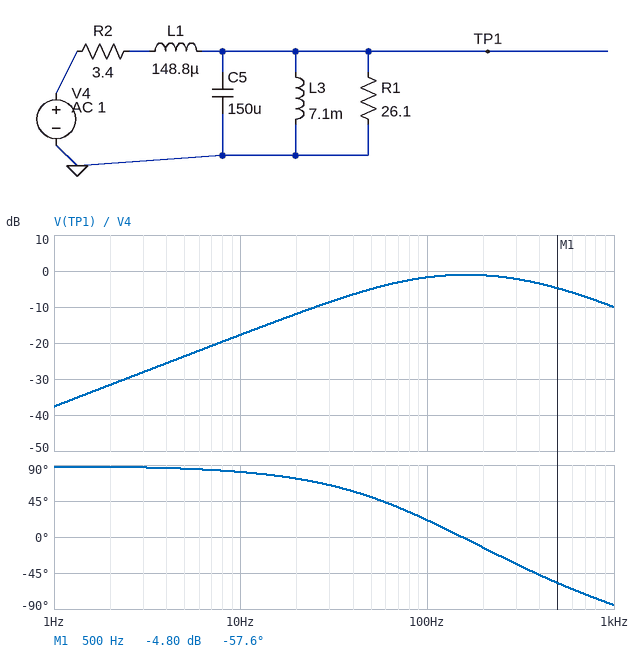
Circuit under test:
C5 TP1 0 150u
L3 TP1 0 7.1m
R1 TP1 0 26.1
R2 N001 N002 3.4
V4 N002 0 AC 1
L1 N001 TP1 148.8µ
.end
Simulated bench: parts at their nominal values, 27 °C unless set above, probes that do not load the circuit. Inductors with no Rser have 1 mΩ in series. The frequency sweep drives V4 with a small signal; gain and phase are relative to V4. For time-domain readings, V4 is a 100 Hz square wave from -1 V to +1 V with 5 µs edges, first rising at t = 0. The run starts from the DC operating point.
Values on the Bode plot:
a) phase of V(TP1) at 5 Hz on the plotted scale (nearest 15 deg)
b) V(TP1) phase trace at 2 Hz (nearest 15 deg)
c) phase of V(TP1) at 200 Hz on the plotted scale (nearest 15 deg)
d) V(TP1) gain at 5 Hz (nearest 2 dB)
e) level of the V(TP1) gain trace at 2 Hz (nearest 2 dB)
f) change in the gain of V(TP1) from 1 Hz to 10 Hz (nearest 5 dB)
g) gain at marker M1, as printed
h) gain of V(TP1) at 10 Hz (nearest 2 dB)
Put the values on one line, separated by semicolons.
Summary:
90 deg; 90 deg; -15 deg; -24 dB; -32 dB; 20 dB; -4.80 dB; -18 dB
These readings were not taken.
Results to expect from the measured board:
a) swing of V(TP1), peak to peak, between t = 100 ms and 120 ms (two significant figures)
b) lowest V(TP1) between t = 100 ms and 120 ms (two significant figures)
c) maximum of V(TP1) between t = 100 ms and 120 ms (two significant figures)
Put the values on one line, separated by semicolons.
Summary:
2.5 V; -1.3 V; 1.3 V
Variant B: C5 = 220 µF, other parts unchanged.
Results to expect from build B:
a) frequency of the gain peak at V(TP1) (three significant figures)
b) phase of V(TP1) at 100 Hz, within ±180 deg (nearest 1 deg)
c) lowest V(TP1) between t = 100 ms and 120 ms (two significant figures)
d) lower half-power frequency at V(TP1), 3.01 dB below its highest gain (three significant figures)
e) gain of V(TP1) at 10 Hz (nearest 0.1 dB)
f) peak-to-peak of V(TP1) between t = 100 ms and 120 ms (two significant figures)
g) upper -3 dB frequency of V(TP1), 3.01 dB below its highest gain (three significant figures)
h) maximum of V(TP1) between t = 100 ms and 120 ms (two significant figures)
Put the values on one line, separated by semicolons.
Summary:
131 Hz; 14 deg; -1.2 V; 55.5 Hz; -17.7 dB; 2.4 V; 310 Hz; 1.2 V
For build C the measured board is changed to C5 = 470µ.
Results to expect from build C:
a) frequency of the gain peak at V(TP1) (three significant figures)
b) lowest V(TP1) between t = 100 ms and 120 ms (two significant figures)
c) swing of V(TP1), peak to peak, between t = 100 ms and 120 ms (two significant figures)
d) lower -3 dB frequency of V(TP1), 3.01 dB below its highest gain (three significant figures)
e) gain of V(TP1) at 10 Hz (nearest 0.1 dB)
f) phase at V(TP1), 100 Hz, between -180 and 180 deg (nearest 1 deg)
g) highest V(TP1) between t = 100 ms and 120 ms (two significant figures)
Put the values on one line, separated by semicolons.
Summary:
88.4 Hz; -1.0 V; 2.1 V; 47.8 Hz; -17.6 dB; -12 deg; 1.0 V
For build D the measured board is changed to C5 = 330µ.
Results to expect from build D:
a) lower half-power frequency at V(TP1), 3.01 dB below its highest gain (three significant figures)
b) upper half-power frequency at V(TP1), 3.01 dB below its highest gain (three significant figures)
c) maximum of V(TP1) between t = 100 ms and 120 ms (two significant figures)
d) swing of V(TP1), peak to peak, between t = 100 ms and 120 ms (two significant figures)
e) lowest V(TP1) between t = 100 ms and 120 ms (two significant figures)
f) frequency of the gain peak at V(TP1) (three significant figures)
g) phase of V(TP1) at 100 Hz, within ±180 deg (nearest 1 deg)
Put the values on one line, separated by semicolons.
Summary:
51.6 Hz; 218 Hz; 1.1 V; 2.3 V; -1.1 V; 106 Hz; 3 deg
